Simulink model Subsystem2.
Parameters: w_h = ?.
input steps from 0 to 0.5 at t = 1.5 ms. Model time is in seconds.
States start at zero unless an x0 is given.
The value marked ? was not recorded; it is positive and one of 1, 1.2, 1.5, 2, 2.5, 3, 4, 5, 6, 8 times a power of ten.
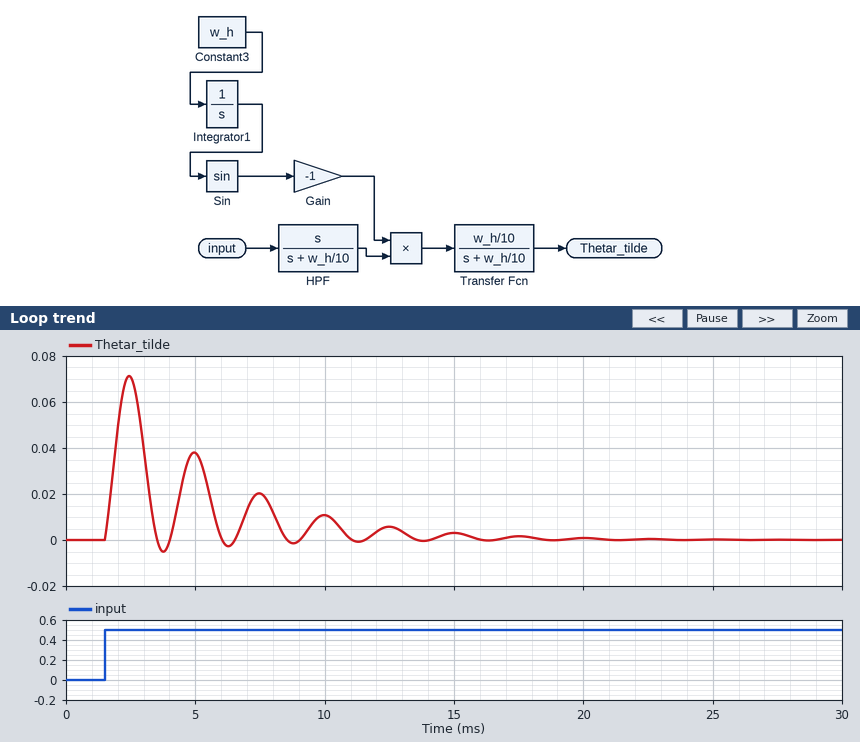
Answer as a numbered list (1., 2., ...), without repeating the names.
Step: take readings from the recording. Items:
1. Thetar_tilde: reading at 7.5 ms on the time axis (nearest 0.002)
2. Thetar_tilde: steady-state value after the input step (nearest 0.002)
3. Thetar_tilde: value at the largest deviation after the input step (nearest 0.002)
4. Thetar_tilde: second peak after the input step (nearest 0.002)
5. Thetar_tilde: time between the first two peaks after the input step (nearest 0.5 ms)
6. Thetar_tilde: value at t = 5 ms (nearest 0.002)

1. 0.020
2. 0.000
3. 0.072
4. 0.038
5. 2.5 ms
6. 0.038
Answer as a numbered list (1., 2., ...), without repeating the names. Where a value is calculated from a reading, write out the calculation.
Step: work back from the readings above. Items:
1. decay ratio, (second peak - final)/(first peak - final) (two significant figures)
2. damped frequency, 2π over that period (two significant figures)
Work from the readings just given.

1. (0.038 - 0) / (0.072 - 0) = 0.53
2. 2π / 2.5 = 2.5 rad/ms
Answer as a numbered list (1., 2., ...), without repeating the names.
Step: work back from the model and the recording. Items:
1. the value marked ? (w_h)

1. 2500
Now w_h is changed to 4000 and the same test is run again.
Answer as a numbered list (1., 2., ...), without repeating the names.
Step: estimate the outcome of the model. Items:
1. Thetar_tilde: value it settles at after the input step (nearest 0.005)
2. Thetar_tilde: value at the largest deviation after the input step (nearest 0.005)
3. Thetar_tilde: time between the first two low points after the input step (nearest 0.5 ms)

1. 0.000
2. -0.070
3. 1.5 ms
